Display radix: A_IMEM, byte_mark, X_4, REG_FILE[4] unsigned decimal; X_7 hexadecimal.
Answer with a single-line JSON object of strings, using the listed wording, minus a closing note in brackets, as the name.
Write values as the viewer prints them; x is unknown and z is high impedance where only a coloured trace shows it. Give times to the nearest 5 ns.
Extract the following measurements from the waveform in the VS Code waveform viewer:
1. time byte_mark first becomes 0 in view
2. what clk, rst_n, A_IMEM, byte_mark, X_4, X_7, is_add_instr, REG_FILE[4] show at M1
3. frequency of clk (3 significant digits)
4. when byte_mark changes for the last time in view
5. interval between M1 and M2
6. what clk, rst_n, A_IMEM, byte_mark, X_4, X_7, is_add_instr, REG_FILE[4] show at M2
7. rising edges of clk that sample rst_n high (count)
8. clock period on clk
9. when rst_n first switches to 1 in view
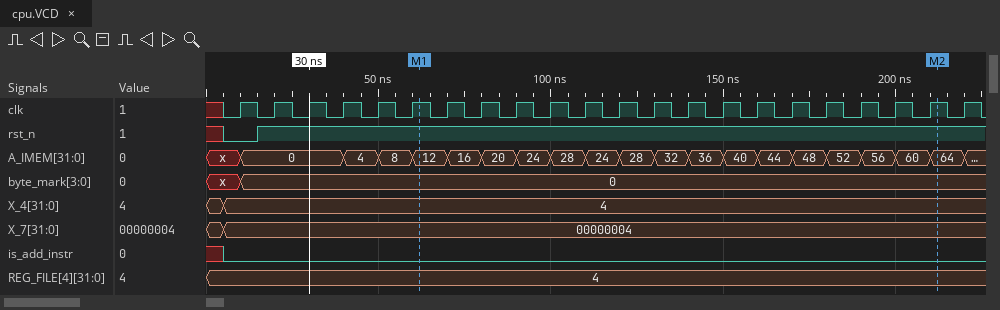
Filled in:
{"time byte_mark first becomes 0 in view": "10 ns", "what clk, rst_n, A_IMEM, byte_mark, X_4, X_7, is_add_instr, REG_FILE[4] show at M1": "clk=1, rst_n=1, A_IMEM=12, byte_mark=0, X_4=4, X_7=00000004, is_add_instr=0, REG_FILE[4]=4", "frequency of clk": "100 MHz", "when byte_mark changes for the last time in view": "10 ns", "interval between M1 and M2": "150 ns", "what clk, rst_n, A_IMEM, byte_mark, X_4, X_7, is_add_instr, REG_FILE[4] show at M2": "clk=1, rst_n=1, A_IMEM=64, byte_mark=0, X_4=4, X_7=00000004, is_add_instr=0, REG_FILE[4]=4", "rising edges of clk that sample rst_n high": "21", "clock period on clk": "10 ns", "when rst_n first switches to 1 in view": "15 ns"}
